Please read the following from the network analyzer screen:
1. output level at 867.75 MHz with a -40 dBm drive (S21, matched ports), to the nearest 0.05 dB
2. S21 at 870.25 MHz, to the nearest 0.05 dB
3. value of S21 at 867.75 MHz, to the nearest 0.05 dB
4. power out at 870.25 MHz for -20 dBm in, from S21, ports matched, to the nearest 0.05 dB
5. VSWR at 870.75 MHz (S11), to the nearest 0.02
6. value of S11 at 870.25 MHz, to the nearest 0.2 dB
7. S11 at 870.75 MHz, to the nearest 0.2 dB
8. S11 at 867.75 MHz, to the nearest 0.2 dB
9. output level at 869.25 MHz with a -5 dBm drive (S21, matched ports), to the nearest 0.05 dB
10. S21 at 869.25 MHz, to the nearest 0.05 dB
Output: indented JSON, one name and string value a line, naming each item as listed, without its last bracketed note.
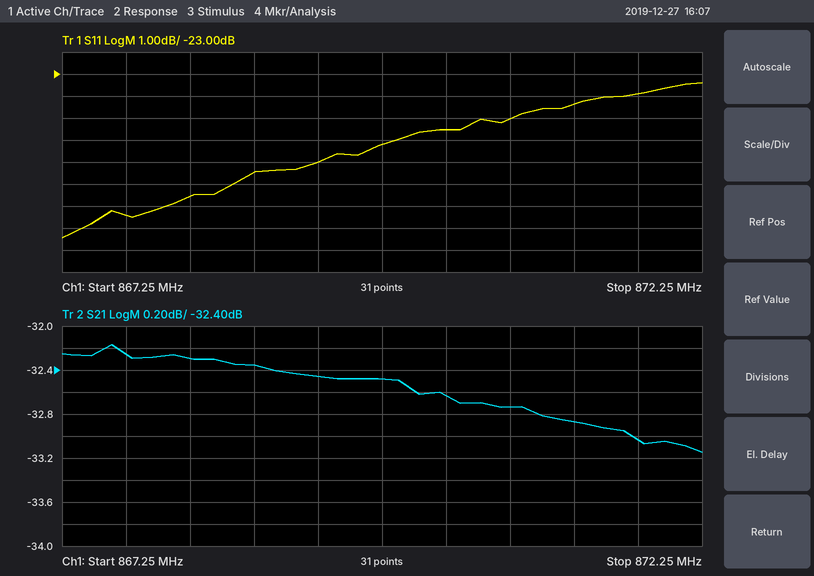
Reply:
{
  "output level at 867.75 MHz with a -40 dBm drive (S21, matched ports), to the nearest 0.05 dB": "-72.25 dBm",
  "S21 at 870.25 MHz, to the nearest 0.05 dB": "-32.65 dB",
  "value of S21 at 867.75 MHz, to the nearest 0.05 dB": "-32.25 dB",
  "power out at 870.25 MHz for -20 dBm in, from S21, ports matched, to the nearest 0.05 dB": "-52.65 dBm",
  "VSWR at 870.75 MHz (S11), to the nearest 0.02": "1.12",
  "value of S11 at 870.25 MHz, to the nearest 0.2 dB": "-25.6 dB",
  "S11 at 870.75 MHz, to the nearest 0.2 dB": "-25.0 dB",
  "S11 at 867.75 MHz, to the nearest 0.2 dB": "-29.4 dB",
  "output level at 869.25 MHz with a -5 dBm drive (S21, matched ports), to the nearest 0.05 dB": "-37.45 dBm",
  "S21 at 869.25 MHz, to the nearest 0.05 dB": "-32.45 dB"
}
